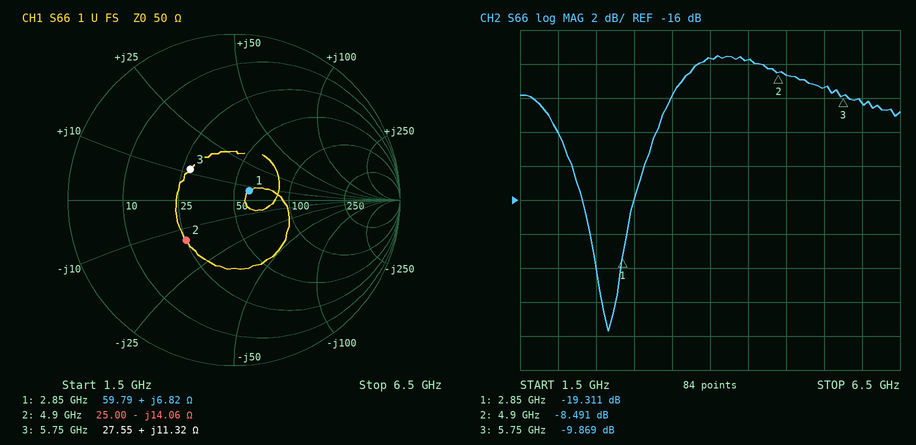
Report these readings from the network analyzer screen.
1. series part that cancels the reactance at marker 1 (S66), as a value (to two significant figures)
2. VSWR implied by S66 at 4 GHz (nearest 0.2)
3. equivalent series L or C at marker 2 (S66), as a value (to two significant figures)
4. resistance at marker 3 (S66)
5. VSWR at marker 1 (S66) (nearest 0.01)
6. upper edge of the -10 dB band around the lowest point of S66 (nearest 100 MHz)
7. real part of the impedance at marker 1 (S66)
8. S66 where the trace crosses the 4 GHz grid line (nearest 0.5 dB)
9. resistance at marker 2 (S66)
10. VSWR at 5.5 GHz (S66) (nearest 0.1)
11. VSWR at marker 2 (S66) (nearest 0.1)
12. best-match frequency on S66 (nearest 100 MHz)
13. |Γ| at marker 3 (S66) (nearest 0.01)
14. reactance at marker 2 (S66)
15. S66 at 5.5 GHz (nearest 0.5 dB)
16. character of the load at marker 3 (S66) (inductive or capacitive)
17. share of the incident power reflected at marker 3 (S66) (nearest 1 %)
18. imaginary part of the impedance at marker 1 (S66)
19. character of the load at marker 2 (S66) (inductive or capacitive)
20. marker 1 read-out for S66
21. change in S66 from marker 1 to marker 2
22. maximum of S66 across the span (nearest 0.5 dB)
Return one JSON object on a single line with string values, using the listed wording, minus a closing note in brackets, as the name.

{"series part that cancels the reactance at marker 1 (S66), as a value": "8.2 pF", "VSWR implied by S66 at 4 GHz": "2.4", "equivalent series L or C at marker 2 (S66), as a value": "2.3 pF", "resistance at marker 3": "27.55 Ω", "VSWR at marker 1 (S66)": "1.24", "upper edge of the -10 dB band around the lowest point of S66": "3.5 GHz", "real part of the impedance at marker 1": "59.79 Ω", "S66 where the trace crosses the 4 GHz grid line": "-7.5 dB", "resistance at marker 2": "25.00 Ω", "VSWR at 5.5 GHz (S66)": "2.0", "VSWR at marker 2 (S66)": "2.2", "best-match frequency on S66": "2.7 GHz", "|Γ| at marker 3 (S66)": "0.32", "reactance at marker 2": "-14.06 Ω", "S66 at 5.5 GHz": "-9.5 dB", "character of the load at marker 3 (S66)": "inductive", "share of the incident power reflected at marker 3 (S66)": "10 %", "imaginary part of the impedance at marker 1": "+6.82 Ω", "character of the load at marker 2 (S66)": "capacitive", "marker 1 read-out for S66": "-19.311 dB", "change in S66 from marker 1 to marker 2": "10.820 dB", "maximum of S66 across the span": "-7.5 dB"}
